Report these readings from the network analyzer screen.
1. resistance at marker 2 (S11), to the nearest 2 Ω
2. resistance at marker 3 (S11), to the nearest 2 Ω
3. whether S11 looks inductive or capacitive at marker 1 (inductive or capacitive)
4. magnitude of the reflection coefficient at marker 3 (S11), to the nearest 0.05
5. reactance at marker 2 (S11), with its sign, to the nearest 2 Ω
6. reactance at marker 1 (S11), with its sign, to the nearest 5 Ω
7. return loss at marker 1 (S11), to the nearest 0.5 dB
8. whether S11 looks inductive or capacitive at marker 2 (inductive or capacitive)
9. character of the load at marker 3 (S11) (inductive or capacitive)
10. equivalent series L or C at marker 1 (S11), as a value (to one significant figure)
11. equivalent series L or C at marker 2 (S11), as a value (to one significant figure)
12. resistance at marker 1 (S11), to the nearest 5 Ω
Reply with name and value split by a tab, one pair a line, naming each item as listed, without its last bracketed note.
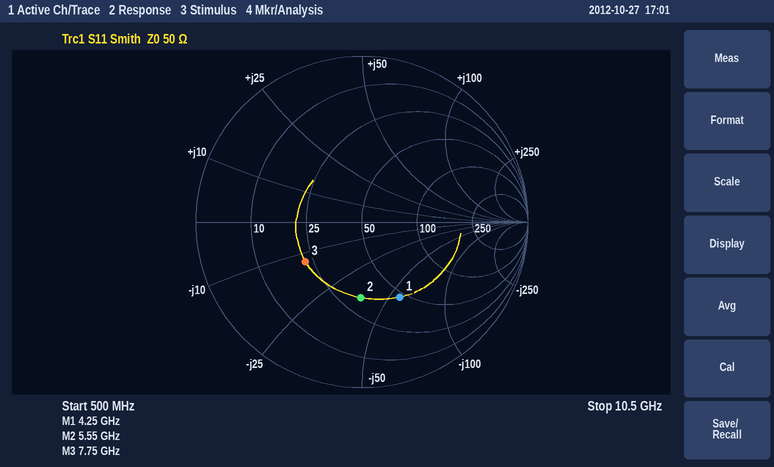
resistance at marker 2 (S11), to the nearest 2 Ω	32 Ω
resistance at marker 3 (S11), to the nearest 2 Ω	22 Ω
whether S11 looks inductive or capacitive at marker 1	capacitive
magnitude of the reflection coefficient at marker 3 (S11), to the nearest 0.05	0.40
reactance at marker 2 (S11), with its sign, to the nearest 2 Ω	-38 Ω
reactance at marker 1 (S11), with its sign, to the nearest 5 Ω	-55 Ω
return loss at marker 1 (S11), to the nearest 0.5 dB	6.0 dB
whether S11 looks inductive or capacitive at marker 2	capacitive
character of the load at marker 3 (S11)	capacitive
equivalent series L or C at marker 1 (S11), as a value	700 fF
equivalent series L or C at marker 2 (S11), as a value	800 fF
resistance at marker 1 (S11), to the nearest 5 Ω	45 Ω
